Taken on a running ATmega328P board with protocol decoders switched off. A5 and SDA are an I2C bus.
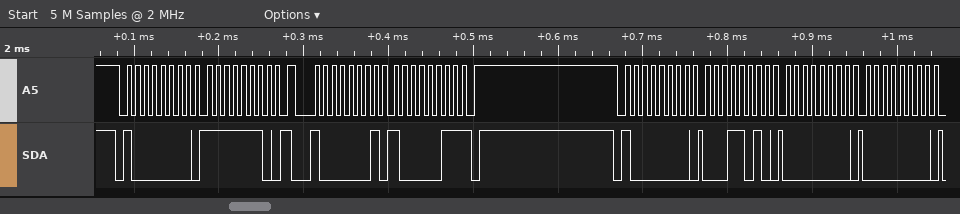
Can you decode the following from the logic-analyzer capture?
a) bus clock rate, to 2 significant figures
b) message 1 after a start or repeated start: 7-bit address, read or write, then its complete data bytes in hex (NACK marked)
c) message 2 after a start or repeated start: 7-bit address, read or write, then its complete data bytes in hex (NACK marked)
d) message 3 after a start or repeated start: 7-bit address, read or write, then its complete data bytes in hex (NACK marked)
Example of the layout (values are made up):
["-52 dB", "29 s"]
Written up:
["100 kHz", "0x40 write: FE", "0x40 read: 83 NACK", "0x40 write: 1A 00 00"]
